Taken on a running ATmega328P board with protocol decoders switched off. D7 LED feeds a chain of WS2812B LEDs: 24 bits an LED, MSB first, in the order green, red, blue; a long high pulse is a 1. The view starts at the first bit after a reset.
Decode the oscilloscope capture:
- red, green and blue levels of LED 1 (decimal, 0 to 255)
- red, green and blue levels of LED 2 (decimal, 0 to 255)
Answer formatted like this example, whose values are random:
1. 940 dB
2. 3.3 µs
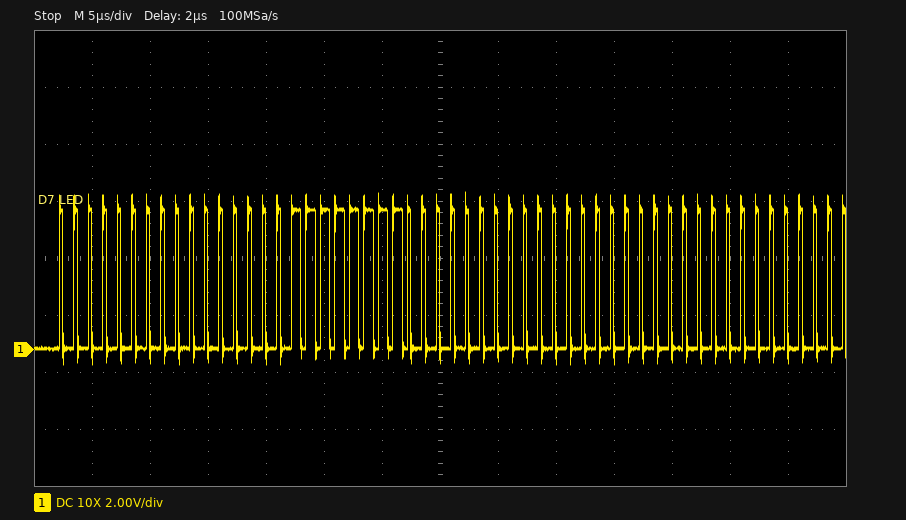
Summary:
1. 0, 0, 255
2. 0, 0, 0
